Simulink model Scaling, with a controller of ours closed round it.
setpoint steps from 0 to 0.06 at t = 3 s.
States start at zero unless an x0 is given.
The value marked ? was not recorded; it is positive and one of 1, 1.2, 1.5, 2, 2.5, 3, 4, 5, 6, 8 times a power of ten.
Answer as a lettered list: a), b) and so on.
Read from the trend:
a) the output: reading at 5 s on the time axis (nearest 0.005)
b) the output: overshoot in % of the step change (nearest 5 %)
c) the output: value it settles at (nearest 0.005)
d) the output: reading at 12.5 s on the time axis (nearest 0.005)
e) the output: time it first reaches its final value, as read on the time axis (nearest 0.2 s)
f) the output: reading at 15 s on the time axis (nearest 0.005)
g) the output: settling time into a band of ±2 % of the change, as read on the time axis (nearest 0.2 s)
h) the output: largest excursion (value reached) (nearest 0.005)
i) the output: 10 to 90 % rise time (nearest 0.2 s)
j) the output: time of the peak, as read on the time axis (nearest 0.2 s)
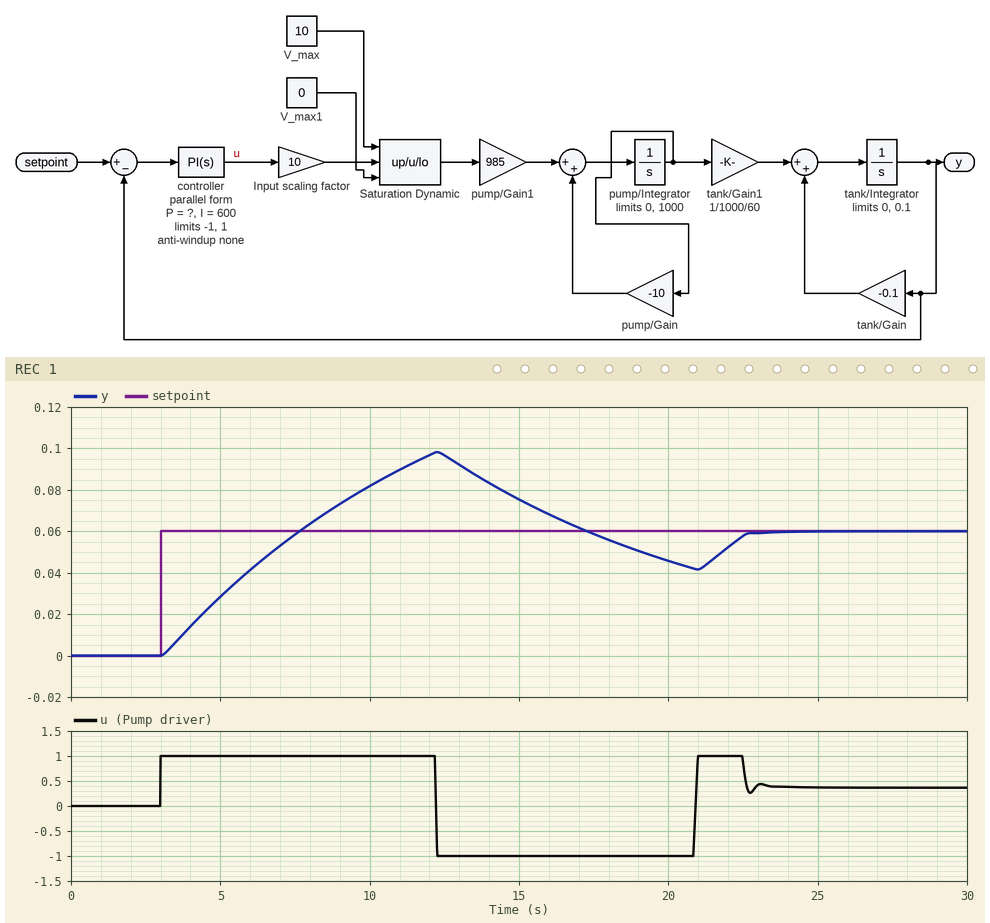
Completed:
a) 0.030
b) 65 %
c) 0.060
d) 0.095
e) 7.6 s
f) 0.075
g) 22.6 s
h) 0.100
i) 3.6 s
j) 12.2 s
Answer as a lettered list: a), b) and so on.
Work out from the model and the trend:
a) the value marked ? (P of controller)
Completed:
a) 600
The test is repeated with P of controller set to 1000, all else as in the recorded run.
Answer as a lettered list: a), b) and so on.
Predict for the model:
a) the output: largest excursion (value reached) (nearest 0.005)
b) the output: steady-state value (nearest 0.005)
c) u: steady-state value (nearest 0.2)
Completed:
a) 0.095
b) 0.060
c) 0.4
